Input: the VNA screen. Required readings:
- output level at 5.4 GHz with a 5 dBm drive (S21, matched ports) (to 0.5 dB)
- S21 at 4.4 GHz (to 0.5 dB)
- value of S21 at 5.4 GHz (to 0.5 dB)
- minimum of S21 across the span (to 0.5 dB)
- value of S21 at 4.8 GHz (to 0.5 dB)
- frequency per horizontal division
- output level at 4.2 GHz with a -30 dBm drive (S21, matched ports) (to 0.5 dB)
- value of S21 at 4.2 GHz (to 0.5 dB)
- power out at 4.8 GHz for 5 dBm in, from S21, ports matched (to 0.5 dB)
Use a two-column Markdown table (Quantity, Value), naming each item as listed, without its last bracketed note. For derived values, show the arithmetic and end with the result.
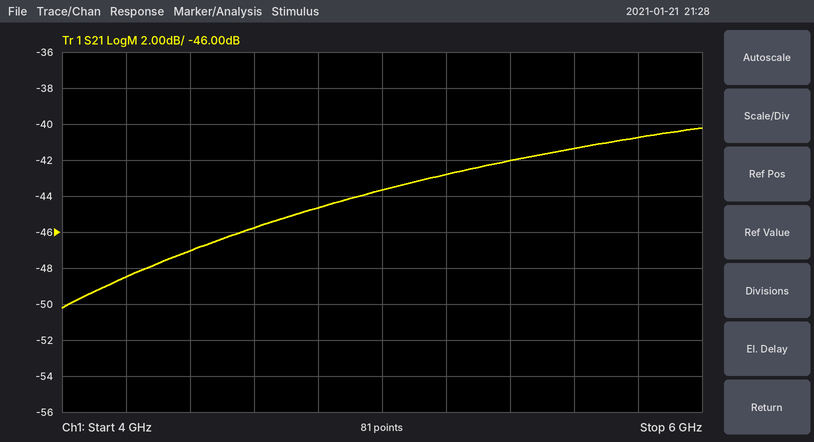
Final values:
| Quantity | Value |
|---|---|
| output level at 5.4 GHz with a 5 dBm drive (S21, matched ports) | 5 dBm + (-42.0 dB) = -37.0 dBm |
| S21 at 4.4 GHz | -47.0 dB |
| value of S21 at 5.4 GHz | -42.0 dB |
| minimum of S21 across the span | -50.0 dB |
| value of S21 at 4.8 GHz | -44.5 dB |
| frequency per horizontal division | 200 MHz |
| output level at 4.2 GHz with a -30 dBm drive (S21, matched ports) | -30 dBm + (-48.5 dB) = -78.5 dBm |
| value of S21 at 4.2 GHz | -48.5 dB |
| power out at 4.8 GHz for 5 dBm in, from S21, ports matched | 5 dBm + (-44.5 dB) = -39.5 dBm |
